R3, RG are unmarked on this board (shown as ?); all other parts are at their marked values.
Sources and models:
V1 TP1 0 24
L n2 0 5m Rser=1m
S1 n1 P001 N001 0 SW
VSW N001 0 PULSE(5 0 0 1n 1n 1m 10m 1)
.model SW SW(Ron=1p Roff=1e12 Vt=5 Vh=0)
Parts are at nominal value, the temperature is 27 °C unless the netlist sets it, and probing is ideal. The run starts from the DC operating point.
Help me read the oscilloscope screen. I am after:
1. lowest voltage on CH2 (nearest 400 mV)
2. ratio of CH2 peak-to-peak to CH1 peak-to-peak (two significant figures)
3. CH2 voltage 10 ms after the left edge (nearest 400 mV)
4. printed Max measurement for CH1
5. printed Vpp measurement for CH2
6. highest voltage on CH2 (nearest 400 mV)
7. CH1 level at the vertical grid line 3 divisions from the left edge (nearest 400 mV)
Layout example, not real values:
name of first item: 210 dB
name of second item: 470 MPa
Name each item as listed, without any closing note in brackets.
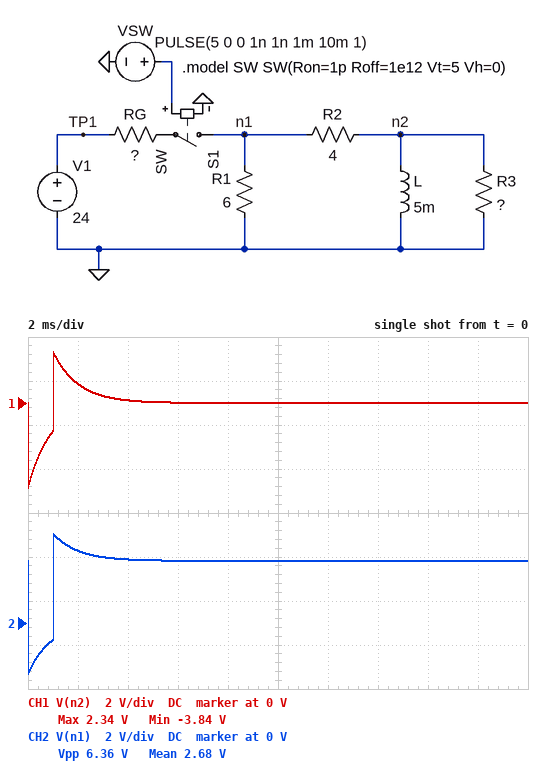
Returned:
lowest voltage on CH2: -2.4 V
ratio of CH2 peak-to-peak to CH1 peak-to-peak: 1.0
CH2 voltage 10 ms after the left edge: 2.8 V
printed Max measurement for CH1: 2.34 V
printed Vpp measurement for CH2: 6.36 V
highest voltage on CH2: 4.0 V
CH1 level at the vertical grid line 3 divisions from the left edge: 0 V
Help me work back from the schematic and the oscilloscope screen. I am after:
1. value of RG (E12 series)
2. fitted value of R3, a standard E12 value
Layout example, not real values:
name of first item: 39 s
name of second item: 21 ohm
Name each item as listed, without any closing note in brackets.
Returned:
value of RG: 18 Ω
fitted value of R3, a standard E12 value: 12 Ω
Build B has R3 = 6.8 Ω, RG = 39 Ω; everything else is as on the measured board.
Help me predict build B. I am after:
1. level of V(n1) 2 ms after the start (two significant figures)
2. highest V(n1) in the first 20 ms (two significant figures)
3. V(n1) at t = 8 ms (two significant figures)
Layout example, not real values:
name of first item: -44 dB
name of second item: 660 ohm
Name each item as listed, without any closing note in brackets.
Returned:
level of V(n1) 2 ms after the start: 1.6 V
highest V(n1) in the first 20 ms: 1.8 V
V(n1) at t = 8 ms: 1.4 V
